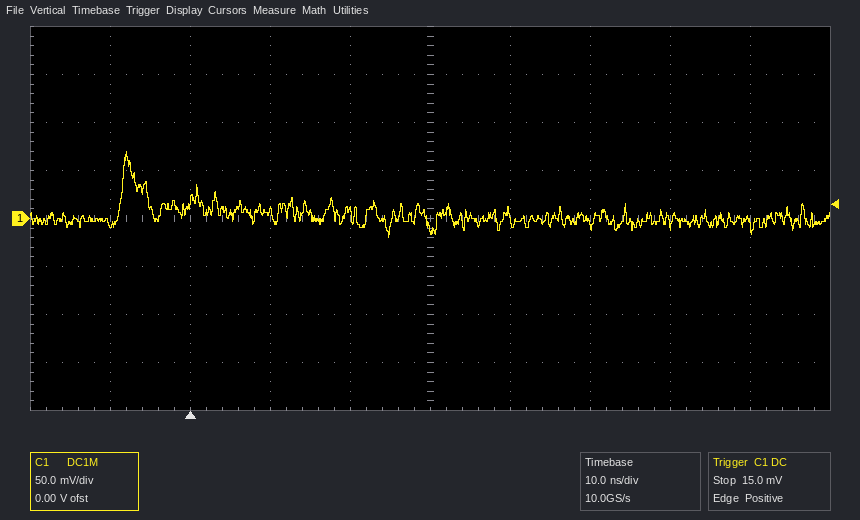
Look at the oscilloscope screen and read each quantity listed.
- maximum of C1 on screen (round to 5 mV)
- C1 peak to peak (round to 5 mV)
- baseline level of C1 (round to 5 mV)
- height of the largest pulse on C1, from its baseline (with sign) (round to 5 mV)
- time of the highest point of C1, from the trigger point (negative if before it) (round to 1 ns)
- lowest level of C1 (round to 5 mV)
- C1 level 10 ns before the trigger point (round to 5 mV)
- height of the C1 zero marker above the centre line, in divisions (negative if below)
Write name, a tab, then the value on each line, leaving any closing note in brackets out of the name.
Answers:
maximum of C1 on screen	70 mV
C1 peak to peak	90 mV
baseline level of C1	0 mV
height of the largest pulse on C1, from its baseline (with sign)	+70 mV
time of the highest point of C1, from the trigger point (negative if before it)	-8 ns
lowest level of C1	-20 mV
C1 level 10 ns before the trigger point	-5 mV
height of the C1 zero marker above the centre line, in divisions	0.0 div
